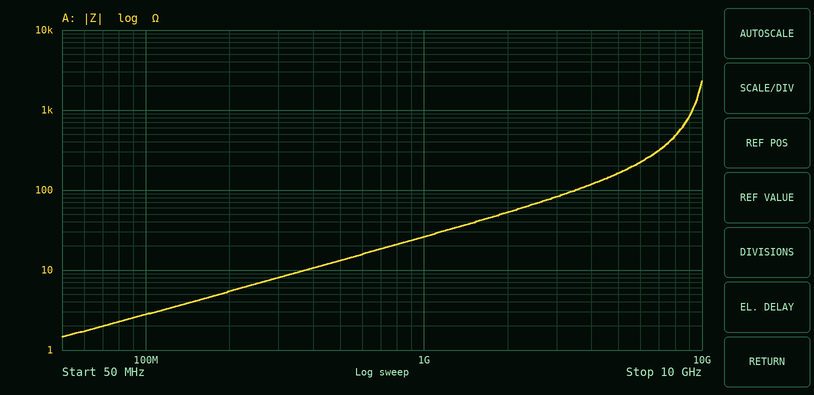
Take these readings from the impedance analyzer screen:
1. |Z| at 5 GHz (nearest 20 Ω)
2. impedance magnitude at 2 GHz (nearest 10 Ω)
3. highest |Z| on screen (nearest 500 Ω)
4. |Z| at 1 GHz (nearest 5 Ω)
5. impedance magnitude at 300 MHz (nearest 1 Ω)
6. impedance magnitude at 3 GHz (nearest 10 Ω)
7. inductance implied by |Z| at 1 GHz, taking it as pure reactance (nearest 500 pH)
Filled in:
160 Ω
50 Ω
2.5 kΩ
25 Ω
8 Ω
80 Ω
4.0 nH
